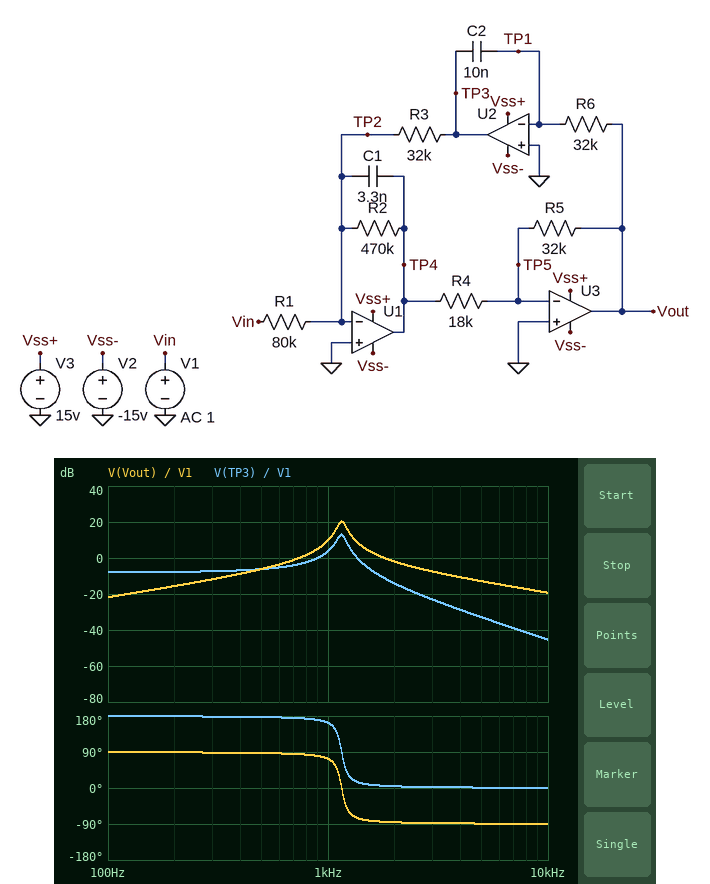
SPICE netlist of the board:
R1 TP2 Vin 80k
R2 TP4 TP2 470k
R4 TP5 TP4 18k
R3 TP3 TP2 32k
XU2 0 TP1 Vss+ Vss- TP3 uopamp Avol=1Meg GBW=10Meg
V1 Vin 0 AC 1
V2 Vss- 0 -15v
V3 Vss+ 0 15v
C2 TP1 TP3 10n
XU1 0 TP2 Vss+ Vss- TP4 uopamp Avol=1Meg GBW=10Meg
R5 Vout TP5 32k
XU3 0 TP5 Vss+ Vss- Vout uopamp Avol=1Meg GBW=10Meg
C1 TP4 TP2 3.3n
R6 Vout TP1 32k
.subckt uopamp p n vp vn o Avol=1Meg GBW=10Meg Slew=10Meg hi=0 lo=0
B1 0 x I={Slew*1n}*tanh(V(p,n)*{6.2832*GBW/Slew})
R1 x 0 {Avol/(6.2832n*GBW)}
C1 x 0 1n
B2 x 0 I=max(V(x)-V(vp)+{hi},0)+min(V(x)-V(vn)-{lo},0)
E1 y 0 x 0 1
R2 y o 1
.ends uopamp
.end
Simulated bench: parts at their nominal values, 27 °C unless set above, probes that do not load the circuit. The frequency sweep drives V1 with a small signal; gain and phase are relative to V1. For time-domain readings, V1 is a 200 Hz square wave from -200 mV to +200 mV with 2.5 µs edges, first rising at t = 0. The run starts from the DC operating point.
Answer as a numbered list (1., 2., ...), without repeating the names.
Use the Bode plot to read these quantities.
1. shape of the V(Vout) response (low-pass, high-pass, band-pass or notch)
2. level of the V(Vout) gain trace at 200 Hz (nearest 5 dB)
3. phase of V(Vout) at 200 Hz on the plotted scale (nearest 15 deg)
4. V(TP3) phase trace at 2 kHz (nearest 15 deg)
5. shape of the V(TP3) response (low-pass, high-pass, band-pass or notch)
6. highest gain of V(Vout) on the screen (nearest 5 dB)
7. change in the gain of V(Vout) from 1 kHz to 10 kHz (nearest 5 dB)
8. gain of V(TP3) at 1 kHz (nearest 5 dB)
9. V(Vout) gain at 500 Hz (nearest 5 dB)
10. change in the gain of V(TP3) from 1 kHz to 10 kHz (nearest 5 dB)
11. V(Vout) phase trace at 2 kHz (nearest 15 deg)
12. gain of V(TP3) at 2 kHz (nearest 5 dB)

1. band-pass
2. -15 dB
3. 90 deg
4. 0 deg
5. low-pass
6. 20 dB
7. -30 dB
8. 5 dB
9. -5 dB
10. -50 dB
11. -90 deg
12. -15 dB
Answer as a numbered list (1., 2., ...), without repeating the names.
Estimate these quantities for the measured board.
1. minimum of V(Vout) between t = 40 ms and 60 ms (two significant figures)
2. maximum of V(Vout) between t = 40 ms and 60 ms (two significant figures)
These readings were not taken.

1. -260 mV
2. 260 mV
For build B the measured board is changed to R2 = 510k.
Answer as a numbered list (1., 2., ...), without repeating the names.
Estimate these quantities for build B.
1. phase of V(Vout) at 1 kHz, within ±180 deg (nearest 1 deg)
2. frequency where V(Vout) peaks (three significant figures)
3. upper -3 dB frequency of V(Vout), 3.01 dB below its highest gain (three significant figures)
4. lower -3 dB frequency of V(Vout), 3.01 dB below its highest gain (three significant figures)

1. 74 deg
2. 1.15 kHz
3. 1.20 kHz
4. 1.11 kHz
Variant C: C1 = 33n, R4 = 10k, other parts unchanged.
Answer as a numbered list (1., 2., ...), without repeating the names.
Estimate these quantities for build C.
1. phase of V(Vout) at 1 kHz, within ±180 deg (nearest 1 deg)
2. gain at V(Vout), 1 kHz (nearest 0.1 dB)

1. -89 deg
2. -11.9 dB
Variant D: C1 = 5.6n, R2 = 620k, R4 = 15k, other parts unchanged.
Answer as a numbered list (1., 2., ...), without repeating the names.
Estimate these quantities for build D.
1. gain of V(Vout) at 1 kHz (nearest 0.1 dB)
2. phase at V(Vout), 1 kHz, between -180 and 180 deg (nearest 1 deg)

1. 20.3 dB
2. -52 deg
